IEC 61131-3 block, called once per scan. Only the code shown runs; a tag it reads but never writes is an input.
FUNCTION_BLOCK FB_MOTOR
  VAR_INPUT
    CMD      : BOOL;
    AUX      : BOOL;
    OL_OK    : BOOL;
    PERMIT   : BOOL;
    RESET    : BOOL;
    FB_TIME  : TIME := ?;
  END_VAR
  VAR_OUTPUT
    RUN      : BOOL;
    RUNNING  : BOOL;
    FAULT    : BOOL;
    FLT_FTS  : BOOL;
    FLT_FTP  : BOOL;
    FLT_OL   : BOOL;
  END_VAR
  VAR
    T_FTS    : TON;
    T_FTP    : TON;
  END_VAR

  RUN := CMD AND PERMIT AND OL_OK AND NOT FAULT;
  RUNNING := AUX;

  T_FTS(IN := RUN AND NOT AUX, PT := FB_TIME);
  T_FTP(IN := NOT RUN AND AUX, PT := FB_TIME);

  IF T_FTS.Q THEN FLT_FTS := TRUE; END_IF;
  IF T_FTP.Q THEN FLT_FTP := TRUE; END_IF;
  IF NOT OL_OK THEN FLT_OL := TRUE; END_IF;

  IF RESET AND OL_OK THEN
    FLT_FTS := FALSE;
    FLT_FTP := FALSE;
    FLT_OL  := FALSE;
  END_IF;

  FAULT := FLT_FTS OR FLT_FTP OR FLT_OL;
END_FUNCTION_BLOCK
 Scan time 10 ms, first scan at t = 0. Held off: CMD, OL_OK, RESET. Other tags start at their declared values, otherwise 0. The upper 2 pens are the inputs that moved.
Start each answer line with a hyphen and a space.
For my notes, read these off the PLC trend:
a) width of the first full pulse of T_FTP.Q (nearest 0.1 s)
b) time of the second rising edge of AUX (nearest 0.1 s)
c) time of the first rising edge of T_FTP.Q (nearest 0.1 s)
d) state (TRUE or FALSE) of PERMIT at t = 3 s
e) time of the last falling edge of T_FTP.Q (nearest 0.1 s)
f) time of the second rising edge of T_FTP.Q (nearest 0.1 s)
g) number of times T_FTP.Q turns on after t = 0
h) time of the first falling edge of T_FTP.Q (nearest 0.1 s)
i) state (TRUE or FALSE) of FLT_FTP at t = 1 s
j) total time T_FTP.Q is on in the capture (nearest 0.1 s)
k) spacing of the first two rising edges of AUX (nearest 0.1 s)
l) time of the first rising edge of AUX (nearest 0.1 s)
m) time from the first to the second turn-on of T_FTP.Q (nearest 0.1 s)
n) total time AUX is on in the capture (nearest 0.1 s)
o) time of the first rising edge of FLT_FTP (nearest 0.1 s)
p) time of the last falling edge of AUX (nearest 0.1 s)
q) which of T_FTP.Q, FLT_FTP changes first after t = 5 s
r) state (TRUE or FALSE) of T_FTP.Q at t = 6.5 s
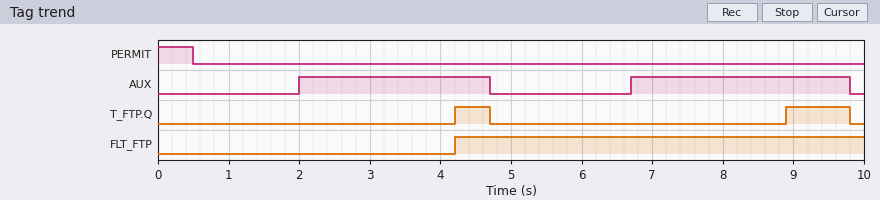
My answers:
- 0.5 s
- 6.7 s
- 4.2 s
- FALSE
- 9.8 s
- 8.9 s
- 2
- 4.7 s
- FALSE
- 1.4 s
- 4.7 s
- 2.0 s
- 4.7 s
- 5.8 s
- 4.2 s
- 9.8 s
- T_FTP.Q
- FALSE
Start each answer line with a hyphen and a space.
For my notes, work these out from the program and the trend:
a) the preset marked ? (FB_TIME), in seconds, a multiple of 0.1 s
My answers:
- 2.2 s
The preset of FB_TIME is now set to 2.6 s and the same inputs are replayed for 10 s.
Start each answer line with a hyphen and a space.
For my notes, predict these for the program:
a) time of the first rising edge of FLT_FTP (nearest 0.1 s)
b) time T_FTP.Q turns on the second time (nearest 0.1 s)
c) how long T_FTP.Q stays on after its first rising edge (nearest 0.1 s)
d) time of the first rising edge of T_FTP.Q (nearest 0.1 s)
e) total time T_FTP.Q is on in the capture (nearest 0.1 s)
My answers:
- 4.6 s
- 9.3 s
- 0.1 s
- 4.6 s
- 0.6 s
